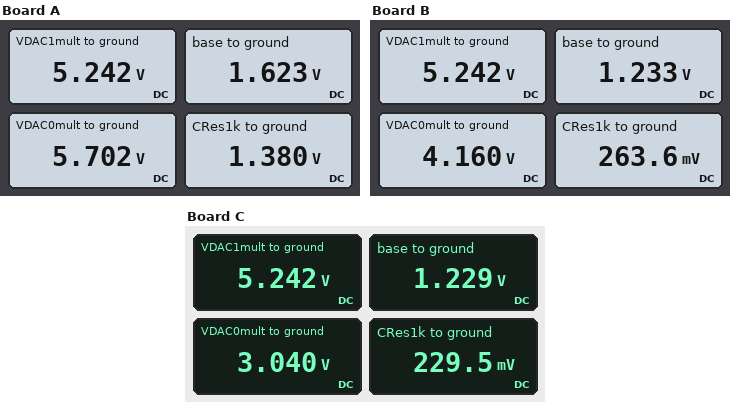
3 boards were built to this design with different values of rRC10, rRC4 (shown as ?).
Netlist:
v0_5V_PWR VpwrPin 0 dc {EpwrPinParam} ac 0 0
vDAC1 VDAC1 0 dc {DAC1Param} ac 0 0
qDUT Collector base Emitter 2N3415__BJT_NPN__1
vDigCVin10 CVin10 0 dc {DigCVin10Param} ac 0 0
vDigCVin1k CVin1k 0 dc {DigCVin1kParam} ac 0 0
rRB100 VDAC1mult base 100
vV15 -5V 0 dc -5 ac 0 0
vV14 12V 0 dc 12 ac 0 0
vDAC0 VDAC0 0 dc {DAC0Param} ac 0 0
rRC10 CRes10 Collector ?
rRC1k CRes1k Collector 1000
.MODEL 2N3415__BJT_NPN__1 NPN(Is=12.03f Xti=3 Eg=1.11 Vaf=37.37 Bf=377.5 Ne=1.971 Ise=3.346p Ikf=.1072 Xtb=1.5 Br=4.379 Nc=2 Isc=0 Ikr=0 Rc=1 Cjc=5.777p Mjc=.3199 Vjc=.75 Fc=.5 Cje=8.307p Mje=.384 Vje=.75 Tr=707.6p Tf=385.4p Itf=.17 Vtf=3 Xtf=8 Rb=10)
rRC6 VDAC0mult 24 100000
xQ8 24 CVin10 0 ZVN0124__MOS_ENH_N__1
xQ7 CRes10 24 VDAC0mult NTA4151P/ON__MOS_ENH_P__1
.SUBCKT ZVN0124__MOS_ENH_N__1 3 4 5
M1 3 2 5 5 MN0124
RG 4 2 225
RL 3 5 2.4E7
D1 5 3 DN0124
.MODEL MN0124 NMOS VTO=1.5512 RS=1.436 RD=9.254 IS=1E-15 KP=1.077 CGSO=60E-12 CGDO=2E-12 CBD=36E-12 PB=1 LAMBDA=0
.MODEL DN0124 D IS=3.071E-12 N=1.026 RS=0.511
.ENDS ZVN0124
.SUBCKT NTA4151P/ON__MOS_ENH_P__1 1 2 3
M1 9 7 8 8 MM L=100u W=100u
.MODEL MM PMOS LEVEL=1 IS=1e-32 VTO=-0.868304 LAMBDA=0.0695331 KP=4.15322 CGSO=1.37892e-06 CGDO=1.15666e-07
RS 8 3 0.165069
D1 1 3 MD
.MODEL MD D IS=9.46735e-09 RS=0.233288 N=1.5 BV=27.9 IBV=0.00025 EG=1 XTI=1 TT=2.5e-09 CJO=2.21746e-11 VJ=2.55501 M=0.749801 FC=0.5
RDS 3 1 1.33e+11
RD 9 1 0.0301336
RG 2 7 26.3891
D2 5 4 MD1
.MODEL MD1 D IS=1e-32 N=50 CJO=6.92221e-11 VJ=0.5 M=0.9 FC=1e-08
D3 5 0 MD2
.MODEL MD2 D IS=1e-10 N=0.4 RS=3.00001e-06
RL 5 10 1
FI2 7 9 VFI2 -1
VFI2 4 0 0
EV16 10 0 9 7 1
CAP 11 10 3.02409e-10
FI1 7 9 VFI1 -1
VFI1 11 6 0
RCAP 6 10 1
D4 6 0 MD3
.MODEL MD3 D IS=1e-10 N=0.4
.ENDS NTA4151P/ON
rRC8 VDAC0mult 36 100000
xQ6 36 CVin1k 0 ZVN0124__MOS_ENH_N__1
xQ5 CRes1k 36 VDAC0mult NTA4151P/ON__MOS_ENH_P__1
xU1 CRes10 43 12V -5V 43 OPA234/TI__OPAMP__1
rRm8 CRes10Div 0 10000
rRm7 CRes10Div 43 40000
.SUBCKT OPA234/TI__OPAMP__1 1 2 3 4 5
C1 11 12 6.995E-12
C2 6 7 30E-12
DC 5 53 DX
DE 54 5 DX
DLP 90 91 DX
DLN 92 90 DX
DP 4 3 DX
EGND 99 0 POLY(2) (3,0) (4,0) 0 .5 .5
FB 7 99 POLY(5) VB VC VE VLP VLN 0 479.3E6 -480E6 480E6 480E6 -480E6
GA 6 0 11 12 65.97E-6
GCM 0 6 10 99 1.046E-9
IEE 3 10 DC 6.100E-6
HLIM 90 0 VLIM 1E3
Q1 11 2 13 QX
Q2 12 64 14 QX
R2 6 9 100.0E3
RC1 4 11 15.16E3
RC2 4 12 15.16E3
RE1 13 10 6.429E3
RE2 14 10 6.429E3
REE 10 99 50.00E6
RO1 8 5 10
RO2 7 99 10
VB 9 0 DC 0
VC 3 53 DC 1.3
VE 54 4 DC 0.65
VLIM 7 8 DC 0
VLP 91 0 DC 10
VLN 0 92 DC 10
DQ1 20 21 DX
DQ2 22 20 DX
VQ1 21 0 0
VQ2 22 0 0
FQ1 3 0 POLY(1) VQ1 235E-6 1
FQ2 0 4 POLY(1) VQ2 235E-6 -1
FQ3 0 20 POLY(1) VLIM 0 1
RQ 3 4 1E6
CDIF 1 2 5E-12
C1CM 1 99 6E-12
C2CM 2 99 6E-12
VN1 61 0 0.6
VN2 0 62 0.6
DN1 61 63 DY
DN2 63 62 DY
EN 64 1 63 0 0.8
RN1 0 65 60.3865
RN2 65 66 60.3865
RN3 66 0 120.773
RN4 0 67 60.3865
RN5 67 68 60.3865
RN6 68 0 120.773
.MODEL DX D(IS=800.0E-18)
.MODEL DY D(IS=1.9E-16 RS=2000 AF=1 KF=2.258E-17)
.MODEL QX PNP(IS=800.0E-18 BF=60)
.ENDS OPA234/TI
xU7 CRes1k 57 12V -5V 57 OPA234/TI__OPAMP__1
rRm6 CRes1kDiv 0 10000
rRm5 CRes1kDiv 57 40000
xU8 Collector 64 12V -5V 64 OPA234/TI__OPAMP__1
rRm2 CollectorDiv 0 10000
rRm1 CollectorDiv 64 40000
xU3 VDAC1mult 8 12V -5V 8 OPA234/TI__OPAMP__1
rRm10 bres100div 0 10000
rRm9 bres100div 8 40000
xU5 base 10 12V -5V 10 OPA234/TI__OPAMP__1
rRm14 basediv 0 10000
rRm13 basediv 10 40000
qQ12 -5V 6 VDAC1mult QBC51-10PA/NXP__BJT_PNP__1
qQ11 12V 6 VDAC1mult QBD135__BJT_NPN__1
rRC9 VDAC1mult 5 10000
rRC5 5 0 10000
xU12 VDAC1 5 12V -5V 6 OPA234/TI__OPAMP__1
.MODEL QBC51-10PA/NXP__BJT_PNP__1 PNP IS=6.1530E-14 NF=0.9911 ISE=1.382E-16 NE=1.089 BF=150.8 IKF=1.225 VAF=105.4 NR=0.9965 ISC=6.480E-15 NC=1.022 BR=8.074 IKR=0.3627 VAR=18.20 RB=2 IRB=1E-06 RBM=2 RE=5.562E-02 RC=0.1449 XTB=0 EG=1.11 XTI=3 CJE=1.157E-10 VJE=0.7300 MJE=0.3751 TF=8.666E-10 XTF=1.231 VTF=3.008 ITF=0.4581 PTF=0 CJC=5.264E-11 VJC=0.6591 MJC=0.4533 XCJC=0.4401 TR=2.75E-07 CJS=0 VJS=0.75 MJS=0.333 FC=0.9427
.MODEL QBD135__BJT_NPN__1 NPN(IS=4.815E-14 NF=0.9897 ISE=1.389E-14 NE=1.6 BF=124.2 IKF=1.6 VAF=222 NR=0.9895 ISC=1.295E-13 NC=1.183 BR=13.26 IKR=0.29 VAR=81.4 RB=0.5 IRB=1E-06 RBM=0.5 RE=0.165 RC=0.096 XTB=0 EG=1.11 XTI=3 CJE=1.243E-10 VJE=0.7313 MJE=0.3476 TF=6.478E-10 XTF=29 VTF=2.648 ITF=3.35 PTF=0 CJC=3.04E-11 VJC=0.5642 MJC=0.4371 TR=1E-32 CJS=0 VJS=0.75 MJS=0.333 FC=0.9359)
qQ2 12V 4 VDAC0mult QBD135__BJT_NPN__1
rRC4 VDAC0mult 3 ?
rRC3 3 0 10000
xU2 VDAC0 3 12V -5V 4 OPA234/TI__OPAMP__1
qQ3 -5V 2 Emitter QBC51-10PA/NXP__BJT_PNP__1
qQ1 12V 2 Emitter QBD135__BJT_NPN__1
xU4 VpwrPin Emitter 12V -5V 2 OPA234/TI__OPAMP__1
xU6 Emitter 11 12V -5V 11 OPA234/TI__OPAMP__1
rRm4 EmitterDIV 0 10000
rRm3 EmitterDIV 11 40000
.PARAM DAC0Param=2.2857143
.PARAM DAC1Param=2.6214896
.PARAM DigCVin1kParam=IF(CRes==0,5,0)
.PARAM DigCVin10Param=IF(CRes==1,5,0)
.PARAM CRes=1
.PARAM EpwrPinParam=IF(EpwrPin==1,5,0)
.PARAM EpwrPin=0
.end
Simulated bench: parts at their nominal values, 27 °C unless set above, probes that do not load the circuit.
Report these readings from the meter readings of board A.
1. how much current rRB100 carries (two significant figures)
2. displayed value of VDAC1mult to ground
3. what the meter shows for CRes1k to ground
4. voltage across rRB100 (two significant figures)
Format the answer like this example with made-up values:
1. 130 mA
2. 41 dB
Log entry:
1. 36 mA
2. 5.242 V
3. 1.380 V
4. 3.6 V
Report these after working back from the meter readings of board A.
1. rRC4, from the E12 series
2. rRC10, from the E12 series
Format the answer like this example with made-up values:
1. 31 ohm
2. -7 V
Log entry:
1. 15 kΩ
2. 4.7 Ω
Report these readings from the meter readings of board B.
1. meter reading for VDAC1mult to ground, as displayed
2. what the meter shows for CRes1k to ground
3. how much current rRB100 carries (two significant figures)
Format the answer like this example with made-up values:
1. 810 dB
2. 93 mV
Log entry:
1. 5.242 V
2. 263.6 mV
3. 40 mA
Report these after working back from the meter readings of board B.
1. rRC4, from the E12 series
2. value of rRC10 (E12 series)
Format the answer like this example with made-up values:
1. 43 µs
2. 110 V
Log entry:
1. 8.2 kΩ
2. 18 Ω
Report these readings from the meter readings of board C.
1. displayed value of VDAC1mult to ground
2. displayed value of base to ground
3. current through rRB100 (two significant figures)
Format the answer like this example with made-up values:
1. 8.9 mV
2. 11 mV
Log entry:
1. 5.242 V
2. 1.229 V
3. 40 mA
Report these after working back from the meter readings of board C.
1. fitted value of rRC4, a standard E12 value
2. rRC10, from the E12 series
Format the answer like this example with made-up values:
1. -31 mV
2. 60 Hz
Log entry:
1. 3.3 kΩ
2. 15 Ω
